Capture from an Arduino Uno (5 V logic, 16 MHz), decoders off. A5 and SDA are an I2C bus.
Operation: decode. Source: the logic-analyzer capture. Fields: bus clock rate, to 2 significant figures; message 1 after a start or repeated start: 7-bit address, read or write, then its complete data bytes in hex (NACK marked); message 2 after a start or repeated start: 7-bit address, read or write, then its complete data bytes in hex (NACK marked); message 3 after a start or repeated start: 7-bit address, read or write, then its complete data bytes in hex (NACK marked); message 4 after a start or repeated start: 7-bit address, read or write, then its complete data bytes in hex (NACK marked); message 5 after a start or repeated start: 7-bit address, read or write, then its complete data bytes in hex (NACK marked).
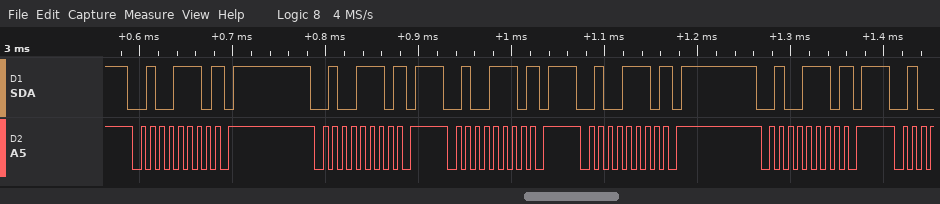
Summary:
100 kHz
0x27 write NACK
0x27 write NACK
0x27 write NACK
0x27 write NACK
0x27 write NACK
